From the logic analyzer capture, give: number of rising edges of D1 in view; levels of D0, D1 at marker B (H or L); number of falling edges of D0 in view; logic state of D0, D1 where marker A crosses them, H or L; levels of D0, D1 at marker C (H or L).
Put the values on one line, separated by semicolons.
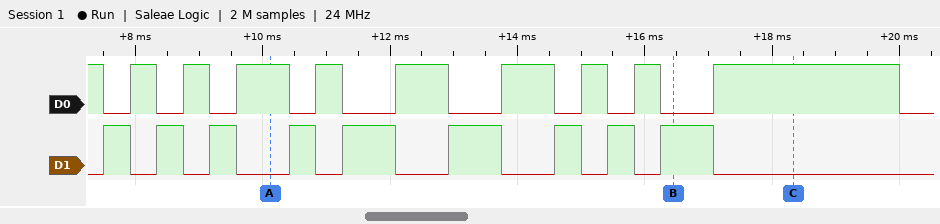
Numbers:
9; D0=L, D1=H; 10; D0=H, D1=L; D0=H, D1=L
